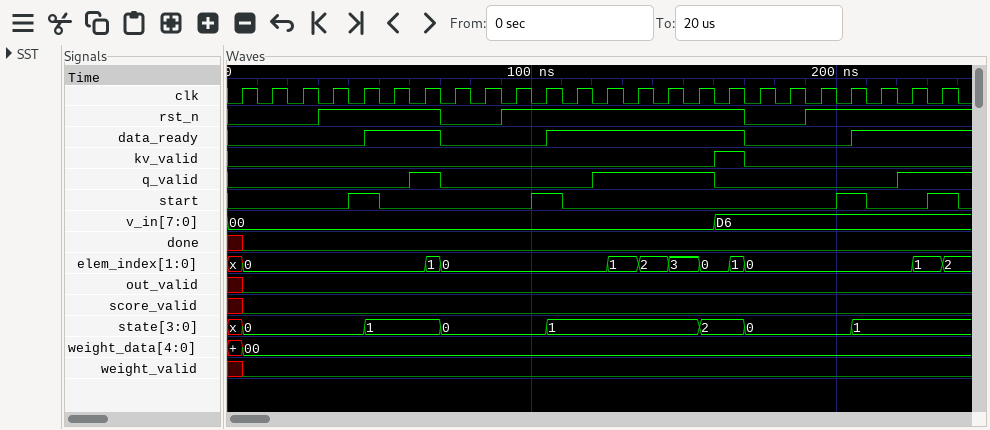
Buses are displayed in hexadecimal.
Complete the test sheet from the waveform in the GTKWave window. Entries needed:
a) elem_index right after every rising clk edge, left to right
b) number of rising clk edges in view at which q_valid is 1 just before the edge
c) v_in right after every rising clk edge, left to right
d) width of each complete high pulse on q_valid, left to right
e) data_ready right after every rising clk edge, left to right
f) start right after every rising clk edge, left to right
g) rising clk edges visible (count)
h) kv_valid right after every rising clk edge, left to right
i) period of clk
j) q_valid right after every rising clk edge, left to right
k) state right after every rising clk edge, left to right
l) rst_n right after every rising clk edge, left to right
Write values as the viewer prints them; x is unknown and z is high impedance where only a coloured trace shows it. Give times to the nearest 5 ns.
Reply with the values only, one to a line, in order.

0, 0, 0, 0, 0, 0, 1, 0, 0, 0, 0, 0, 1, 2, 3, 0, 1, 0, 0, 0, 0, 0, 1, 2
7
00, 00, 00, 00, 00, 00, 00, 00, 00, 00, 00, 00, 00, 00, 00, 00, D6, D6, D6, D6, D6, D6, D6, D6
10 ns, 40 ns
0 0 0 0 1 1 1 0 0 0 1 1 1 1 1 1 1 0 0 0 1 1 1 1
0 0 0 0 1 0 0 0 0 0 1 0 0 0 0 0 0 0 0 0 1 0 0 1
24
0 0 0 0 0 0 0 0 0 0 0 0 0 0 0 0 1 0 0 0 0 0 0 0
10 ns
0 0 0 0 0 0 1 0 0 0 0 0 1 1 1 1 0 0 0 0 0 0 1 1
0, 0, 0, 0, 1, 1, 1, 0, 0, 0, 1, 1, 1, 1, 1, 2, 2, 0, 0, 0, 1, 1, 1, 1
0 0 0 1 1 1 1 0 0 1 1 1 1 1 1 1 1 0 0 1 1 1 1 1
